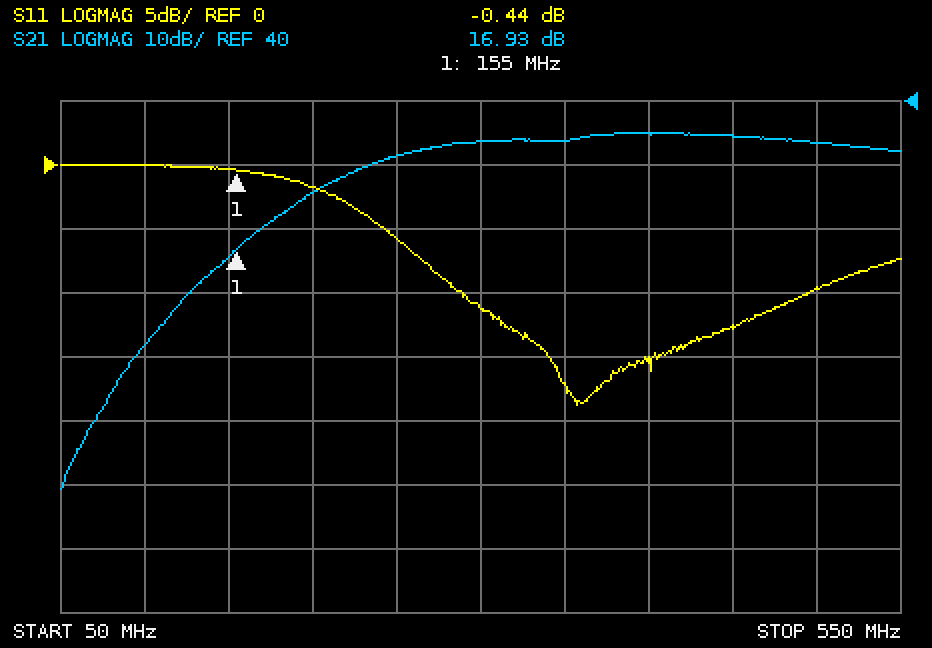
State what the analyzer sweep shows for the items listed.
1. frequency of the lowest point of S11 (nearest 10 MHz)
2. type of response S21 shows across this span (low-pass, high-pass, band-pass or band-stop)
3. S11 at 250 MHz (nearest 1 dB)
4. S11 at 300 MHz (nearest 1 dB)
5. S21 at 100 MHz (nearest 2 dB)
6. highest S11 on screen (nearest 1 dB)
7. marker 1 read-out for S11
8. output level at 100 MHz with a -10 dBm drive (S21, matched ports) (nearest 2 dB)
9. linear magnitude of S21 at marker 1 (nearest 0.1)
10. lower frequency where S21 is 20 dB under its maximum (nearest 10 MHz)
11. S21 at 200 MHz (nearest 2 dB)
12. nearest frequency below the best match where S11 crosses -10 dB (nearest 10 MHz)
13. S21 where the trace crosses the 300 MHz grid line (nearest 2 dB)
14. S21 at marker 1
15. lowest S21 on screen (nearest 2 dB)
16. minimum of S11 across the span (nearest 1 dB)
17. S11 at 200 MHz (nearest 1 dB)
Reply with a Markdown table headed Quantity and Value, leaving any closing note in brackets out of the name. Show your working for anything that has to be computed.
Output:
| Quantity | Value |
|---|---|
| frequency of the lowest point of S11 | 360 MHz |
| type of response S21 shows across this span | high-pass |
| S11 at 250 MHz | -6 dB |
| S11 at 300 MHz | -11 dB |
| S21 at 100 MHz | 2 dB |
| highest S11 on screen | 0 dB |
| marker 1 read-out for S11 | -0.44 dB |
| output level at 100 MHz with a -10 dBm drive (S21, matched ports) | -10 dBm + (2 dB) = -8 dBm |
| linear magnitude of S21 at marker 1 | 10^(16.93/20) ≈ 7.0 |
| lower frequency where S21 is 20 dB under its maximum | 150 MHz |
| S21 at 200 MHz | 26 dB |
| nearest frequency below the best match where S11 crosses -10 dB | 290 MHz |
| S21 where the trace crosses the 300 MHz grid line | 34 dB |
| S21 at marker 1 | 16.93 dB |
| lowest S21 on screen | -20 dB |
| minimum of S11 across the span | -19 dB |
| S11 at 200 MHz | -2 dB |
